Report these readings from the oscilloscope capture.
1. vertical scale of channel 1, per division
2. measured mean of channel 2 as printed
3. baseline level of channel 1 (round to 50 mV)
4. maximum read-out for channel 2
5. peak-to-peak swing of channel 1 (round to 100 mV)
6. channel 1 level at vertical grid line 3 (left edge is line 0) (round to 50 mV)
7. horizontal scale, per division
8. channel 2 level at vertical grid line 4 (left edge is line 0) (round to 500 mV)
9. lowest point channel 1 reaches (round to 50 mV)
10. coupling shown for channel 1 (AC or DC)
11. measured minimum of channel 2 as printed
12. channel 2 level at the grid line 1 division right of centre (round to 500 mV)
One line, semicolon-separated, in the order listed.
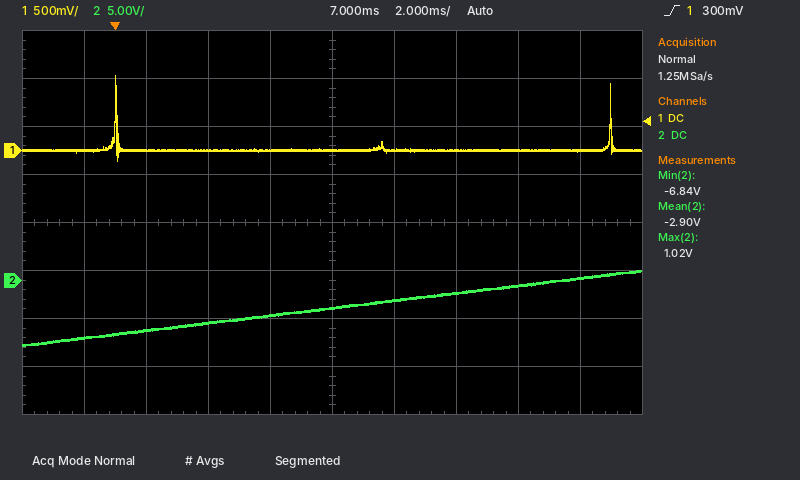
500 mV; -2.90 V; 0 mV; 1.02 V; 900 mV; 0 mV; 2 ms; -3.5 V; -100 mV; DC; -6.84 V; -2.0 V
